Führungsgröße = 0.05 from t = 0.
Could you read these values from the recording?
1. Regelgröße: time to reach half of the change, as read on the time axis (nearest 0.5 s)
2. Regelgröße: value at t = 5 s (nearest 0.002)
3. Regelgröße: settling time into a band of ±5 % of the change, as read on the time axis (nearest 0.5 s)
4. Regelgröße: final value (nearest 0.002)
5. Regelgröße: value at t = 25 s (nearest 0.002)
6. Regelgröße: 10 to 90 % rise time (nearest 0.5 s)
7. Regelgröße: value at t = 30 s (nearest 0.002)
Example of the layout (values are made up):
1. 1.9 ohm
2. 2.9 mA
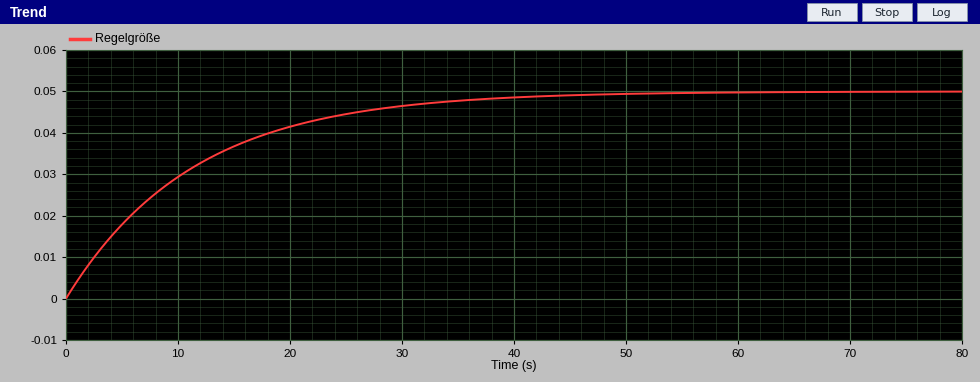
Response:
1. 8.0 s
2. 0.018
3. 34.0 s
4. 0.050
5. 0.044
6. 25.0 s
7. 0.046
